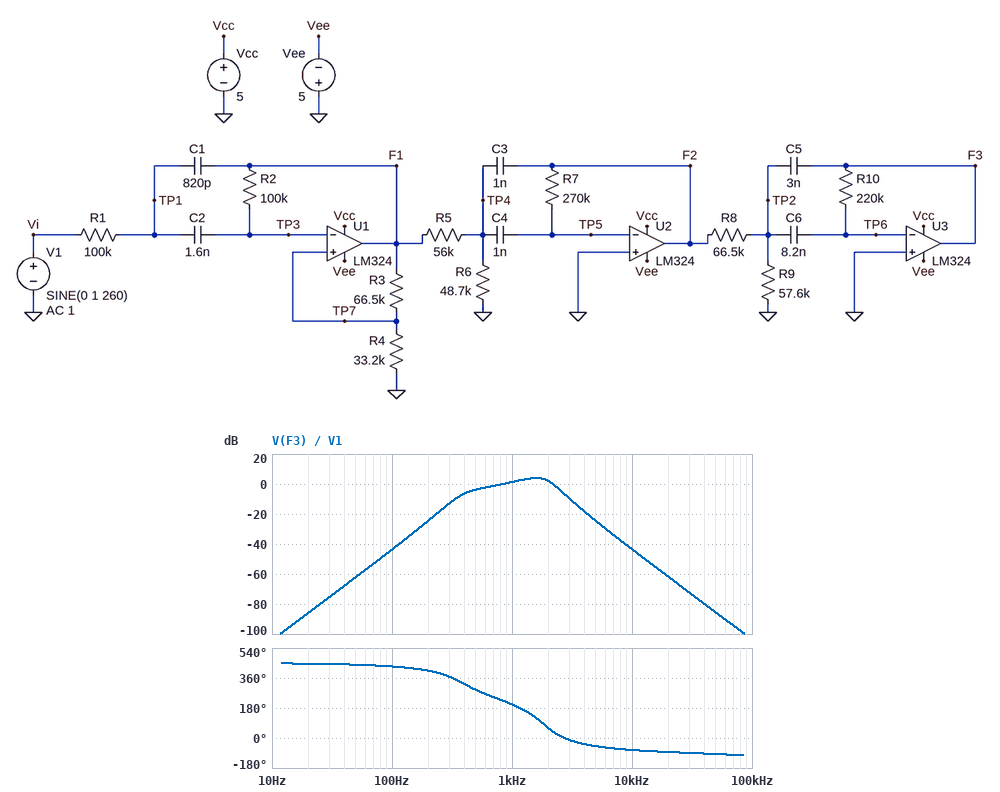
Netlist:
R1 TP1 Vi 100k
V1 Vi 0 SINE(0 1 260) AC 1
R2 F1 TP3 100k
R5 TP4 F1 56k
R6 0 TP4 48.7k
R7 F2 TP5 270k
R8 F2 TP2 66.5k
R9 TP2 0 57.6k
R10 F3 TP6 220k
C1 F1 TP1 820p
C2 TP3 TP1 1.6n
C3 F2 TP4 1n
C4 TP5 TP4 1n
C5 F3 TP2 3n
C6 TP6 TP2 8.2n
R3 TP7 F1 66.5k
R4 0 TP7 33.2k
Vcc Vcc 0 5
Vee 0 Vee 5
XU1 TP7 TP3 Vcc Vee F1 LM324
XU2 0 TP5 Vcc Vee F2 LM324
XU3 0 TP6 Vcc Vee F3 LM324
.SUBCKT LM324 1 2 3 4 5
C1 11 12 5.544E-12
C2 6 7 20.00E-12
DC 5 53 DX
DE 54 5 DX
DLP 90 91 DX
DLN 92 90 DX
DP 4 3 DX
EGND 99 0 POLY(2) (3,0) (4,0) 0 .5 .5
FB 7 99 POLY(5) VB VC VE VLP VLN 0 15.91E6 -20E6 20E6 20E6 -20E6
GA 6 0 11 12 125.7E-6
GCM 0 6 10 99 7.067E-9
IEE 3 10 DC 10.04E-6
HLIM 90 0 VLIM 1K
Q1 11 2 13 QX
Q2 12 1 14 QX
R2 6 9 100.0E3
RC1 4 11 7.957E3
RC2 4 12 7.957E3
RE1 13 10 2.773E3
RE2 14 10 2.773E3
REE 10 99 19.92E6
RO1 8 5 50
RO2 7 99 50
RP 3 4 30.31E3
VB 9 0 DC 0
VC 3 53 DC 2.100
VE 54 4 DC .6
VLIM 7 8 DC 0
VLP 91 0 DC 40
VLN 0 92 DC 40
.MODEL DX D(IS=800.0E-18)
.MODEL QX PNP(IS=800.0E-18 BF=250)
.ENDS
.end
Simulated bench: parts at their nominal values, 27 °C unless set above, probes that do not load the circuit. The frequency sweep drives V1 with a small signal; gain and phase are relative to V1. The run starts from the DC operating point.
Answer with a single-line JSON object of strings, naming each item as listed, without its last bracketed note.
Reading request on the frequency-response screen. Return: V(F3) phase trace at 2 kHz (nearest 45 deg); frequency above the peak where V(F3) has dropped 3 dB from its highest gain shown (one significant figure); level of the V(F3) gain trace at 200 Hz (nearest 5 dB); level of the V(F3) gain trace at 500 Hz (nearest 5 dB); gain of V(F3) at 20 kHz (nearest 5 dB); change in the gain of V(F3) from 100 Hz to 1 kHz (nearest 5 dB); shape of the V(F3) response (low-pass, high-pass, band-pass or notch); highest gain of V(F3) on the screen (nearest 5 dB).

{"V(F3) phase trace at 2 kHz": "45 deg", "frequency above the peak where V(F3) has dropped 3 dB from its highest gain shown": "2 kHz", "level of the V(F3) gain trace at 200 Hz": "-25 dB", "level of the V(F3) gain trace at 500 Hz": "-5 dB", "gain of V(F3) at 20 kHz": "-60 dB", "change in the gain of V(F3) from 100 Hz to 1 kHz": "45 dB", "shape of the V(F3) response": "band-pass", "highest gain of V(F3) on the screen": "5 dB"}
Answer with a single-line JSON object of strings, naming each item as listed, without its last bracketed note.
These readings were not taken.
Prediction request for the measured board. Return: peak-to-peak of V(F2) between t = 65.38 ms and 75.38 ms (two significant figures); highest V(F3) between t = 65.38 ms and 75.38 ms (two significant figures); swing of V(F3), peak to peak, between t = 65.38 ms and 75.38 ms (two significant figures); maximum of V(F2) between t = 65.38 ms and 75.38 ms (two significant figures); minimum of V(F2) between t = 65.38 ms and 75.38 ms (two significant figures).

{"peak-to-peak of V(F2) between t = 65.38 ms and 75.38 ms": "160 mV", "highest V(F3) between t = 65.38 ms and 75.38 ms": "140 mV", "swing of V(F3), peak to peak, between t = 65.38 ms and 75.38 ms": "280 mV", "maximum of V(F2) between t = 65.38 ms and 75.38 ms": "76 mV", "minimum of V(F2) between t = 65.38 ms and 75.38 ms": "-87 mV"}
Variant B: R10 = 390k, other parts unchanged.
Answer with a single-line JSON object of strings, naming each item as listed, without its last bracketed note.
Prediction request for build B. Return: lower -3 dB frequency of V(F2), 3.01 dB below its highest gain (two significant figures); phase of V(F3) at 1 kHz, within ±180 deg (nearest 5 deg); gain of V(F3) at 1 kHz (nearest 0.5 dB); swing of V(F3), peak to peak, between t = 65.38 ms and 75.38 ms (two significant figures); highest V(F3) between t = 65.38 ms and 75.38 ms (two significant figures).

{"lower -3 dB frequency of V(F2), 3.01 dB below its highest gain": "1.3 kHz", "phase of V(F3) at 1 kHz, within ±180 deg": "-170 deg", "gain of V(F3) at 1 kHz": "1.0 dB", "swing of V(F3), peak to peak, between t = 65.38 ms and 75.38 ms": "660 mV", "highest V(F3) between t = 65.38 ms and 75.38 ms": "320 mV"}
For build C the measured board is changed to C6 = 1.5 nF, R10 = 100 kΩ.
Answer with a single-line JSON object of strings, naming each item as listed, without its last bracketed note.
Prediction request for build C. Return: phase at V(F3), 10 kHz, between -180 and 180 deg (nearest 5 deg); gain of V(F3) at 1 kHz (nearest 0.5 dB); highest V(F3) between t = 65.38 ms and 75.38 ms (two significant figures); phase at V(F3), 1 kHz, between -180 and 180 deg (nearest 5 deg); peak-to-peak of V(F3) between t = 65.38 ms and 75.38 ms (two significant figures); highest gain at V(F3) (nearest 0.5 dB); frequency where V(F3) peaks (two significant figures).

{"phase at V(F3), 10 kHz, between -180 and 180 deg": "-65 deg", "gain of V(F3) at 1 kHz": "-4.5 dB", "highest V(F3) between t = 65.38 ms and 75.38 ms": "7.4 mV", "phase at V(F3), 1 kHz, between -180 and 180 deg": "-60 deg", "peak-to-peak of V(F3) between t = 65.38 ms and 75.38 ms": "19 mV", "highest gain at V(F3)": "3.5 dB", "frequency where V(F3) peaks": "1.7 kHz"}
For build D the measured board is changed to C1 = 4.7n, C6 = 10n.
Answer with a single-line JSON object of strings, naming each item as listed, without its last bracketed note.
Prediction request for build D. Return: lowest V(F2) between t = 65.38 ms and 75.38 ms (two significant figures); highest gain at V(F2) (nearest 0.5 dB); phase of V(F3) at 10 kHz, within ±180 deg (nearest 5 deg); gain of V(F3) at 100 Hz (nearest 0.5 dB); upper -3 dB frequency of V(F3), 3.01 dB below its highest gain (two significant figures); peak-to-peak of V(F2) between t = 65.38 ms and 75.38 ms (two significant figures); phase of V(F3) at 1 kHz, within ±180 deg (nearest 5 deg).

{"lowest V(F2) between t = 65.38 ms and 75.38 ms": "-73 mV", "highest gain at V(F2)": "-4.5 dB", "phase of V(F3) at 10 kHz, within ±180 deg": "-75 deg", "gain of V(F3) at 100 Hz": "-42.0 dB", "upper -3 dB frequency of V(F3), 3.01 dB below its highest gain": "1.9 kHz", "peak-to-peak of V(F2) between t = 65.38 ms and 75.38 ms": "140 mV", "phase of V(F3) at 1 kHz, within ±180 deg": "145 deg"}
